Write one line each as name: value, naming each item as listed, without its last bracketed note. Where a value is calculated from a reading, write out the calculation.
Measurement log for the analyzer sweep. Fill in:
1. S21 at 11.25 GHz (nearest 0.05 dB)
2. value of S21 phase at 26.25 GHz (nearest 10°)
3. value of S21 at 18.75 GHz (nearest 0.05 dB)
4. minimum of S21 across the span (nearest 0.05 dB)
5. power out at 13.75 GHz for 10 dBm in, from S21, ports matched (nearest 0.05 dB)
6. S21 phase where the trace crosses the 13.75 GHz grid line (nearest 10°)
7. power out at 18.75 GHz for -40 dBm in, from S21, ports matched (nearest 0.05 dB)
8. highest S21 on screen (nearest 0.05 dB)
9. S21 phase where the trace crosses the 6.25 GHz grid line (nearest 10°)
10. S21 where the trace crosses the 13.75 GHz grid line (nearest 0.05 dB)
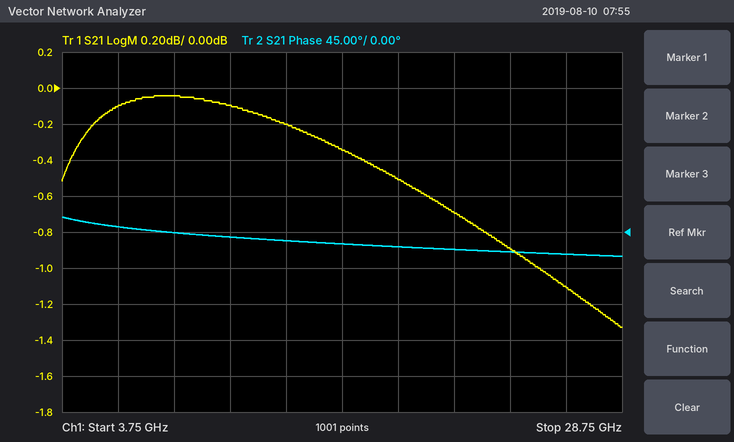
S21 at 11.25 GHz: -0.10 dB
value of S21 phase at 26.25 GHz: -30°
value of S21 at 18.75 GHz: -0.50 dB
minimum of S21 across the span: -1.35 dB
power out at 13.75 GHz for 10 dBm in, from S21, ports matched: 10 dBm + (-0.20 dB) = 9.80 dBm
S21 phase where the trace crosses the 13.75 GHz grid line: -10°
power out at 18.75 GHz for -40 dBm in, from S21, ports matched: -40 dBm + (-0.50 dB) = -40.50 dBm
highest S21 on screen: -0.05 dB
S21 phase where the trace crosses the 6.25 GHz grid line: 10°
S21 where the trace crosses the 13.75 GHz grid line: -0.20 dB
